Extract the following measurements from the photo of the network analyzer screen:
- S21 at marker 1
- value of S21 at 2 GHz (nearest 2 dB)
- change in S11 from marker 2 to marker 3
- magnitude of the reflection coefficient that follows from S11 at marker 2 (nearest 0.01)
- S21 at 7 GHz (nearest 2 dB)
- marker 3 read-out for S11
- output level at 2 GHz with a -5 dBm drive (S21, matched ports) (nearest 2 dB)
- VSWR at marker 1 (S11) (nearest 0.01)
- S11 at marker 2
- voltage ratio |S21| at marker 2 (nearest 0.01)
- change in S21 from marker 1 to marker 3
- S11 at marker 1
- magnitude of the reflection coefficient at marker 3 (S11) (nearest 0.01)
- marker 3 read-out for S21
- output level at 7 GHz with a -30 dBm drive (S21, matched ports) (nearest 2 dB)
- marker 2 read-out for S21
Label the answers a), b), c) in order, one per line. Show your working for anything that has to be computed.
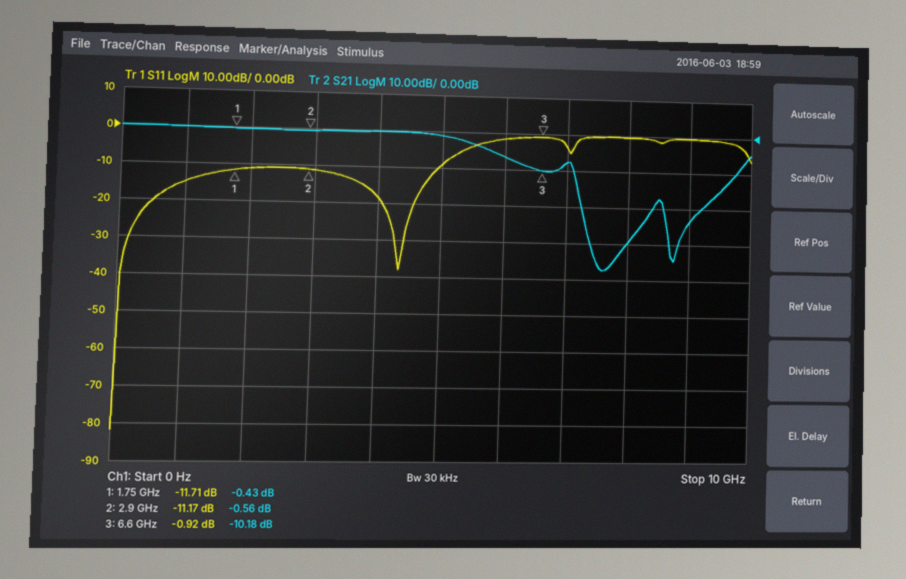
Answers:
a) -0.43 dB
b) 0 dB
c) -0.92 − (-11.17) = 10.25 dB
d) 10^(-11.17/20) ≈ 0.28
e) -8 dB
f) -0.92 dB
g) -5 dBm + (0 dB) = -6 dBm
h) (1 + 0.2597)/(1 − 0.2597) ≈ 1.70
i) -11.17 dB
j) 10^(-0.56/20) ≈ 0.94
k) -10.18 − (-0.43) = -9.75 dB
l) -11.71 dB
m) 10^(-0.92/20) ≈ 0.90
n) -10.18 dB
o) -30 dBm + (-8 dB) = -38 dBm
p) -0.56 dB
